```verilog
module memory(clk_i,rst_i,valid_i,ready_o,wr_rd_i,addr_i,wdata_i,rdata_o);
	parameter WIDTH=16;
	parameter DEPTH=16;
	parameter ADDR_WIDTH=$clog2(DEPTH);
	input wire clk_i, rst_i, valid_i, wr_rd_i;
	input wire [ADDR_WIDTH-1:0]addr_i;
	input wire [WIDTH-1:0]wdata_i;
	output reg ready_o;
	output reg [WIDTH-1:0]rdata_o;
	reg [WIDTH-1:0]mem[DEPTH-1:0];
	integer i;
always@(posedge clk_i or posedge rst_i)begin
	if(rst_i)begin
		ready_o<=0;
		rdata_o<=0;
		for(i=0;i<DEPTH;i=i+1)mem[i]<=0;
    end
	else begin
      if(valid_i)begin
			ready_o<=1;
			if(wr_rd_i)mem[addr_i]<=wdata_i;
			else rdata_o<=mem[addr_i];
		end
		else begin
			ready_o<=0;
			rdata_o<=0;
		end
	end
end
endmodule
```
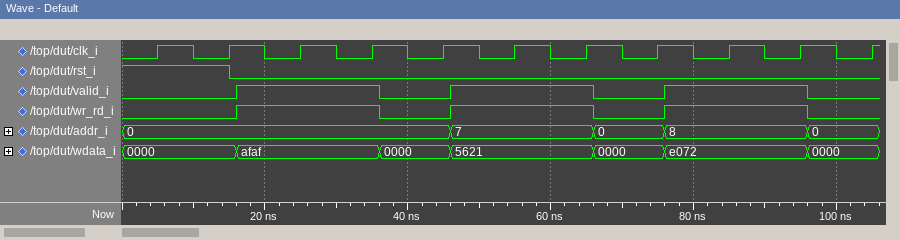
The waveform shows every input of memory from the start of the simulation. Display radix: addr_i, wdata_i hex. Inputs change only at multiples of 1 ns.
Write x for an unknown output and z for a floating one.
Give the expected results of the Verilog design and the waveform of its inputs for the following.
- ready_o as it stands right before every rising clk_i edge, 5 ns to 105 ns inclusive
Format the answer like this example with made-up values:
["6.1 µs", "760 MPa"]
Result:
["0 0 0 1 1 0 1 1 0 1 1"]
